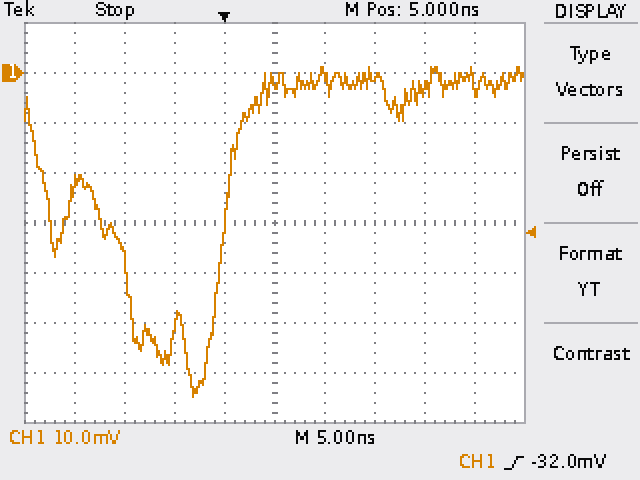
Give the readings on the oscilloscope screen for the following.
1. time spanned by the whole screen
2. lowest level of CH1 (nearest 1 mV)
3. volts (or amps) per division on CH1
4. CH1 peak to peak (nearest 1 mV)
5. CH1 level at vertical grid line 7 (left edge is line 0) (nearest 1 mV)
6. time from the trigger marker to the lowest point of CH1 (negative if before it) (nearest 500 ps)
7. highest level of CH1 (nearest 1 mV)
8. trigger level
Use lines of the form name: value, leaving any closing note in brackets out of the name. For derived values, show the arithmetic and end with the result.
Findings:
time spanned by the whole screen: 50 ns
lowest level of CH1: -65 mV
volts (or amps) per division on CH1: 10 mV
CH1 peak to peak: 1 mV − (-65 mV) = 66 mV
CH1 level at vertical grid line 7 (left edge is line 0): -1 mV
time from the trigger marker to the lowest point of CH1 (negative if before it): -3.0 ns
highest level of CH1: 1 mV
trigger level: -32.0 mV
